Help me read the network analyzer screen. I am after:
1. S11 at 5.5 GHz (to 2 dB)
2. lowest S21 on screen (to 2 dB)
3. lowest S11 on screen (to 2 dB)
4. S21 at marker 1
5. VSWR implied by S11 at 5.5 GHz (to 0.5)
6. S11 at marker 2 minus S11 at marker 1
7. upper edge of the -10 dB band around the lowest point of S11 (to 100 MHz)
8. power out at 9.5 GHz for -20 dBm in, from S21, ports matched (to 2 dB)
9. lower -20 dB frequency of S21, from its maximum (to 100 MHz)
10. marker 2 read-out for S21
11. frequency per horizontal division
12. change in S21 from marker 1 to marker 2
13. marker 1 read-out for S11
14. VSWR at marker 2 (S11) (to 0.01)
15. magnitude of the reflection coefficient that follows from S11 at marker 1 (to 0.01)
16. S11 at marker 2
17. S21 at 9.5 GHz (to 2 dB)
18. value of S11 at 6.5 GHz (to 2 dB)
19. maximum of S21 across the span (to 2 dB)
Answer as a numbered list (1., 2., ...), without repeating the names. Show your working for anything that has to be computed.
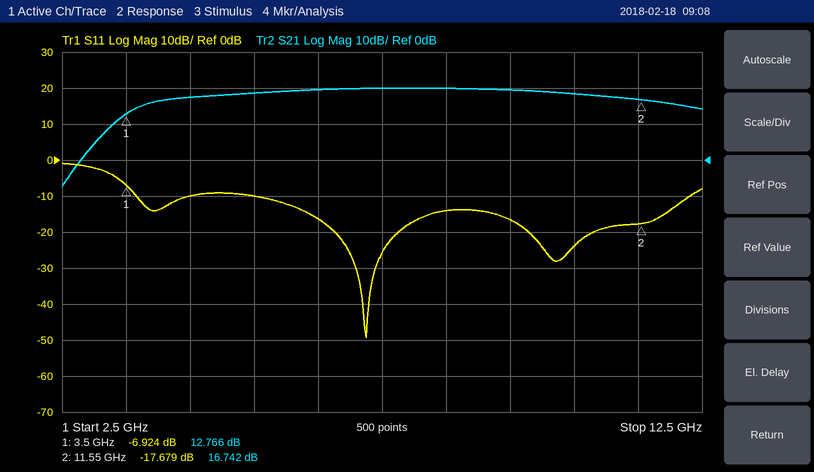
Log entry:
1. -10 dB
2. -8 dB
3. -50 dB
4. 12.766 dB
5. |Γ| = 10^(-10/20) = 0.3162; VSWR = (1 + 0.3162)/(1 − 0.3162) ≈ 1.92, so 2.0 to the nearest 0.5
6. -17.679 − (-6.924) = -10.755 dB
7. 12.3 GHz
8. -20 dBm + (20 dB) = 0 dBm
9. 2.8 GHz
10. 16.742 dB
11. 1 GHz
12. 16.742 − (12.766) = 3.976 dB
13. -6.924 dB
14. (1 + 0.1306)/(1 − 0.1306) ≈ 1.30
15. 10^(-6.924/20) ≈ 0.45
16. -17.679 dB
17. 20 dB
18. -16 dB
19. 20 dB
